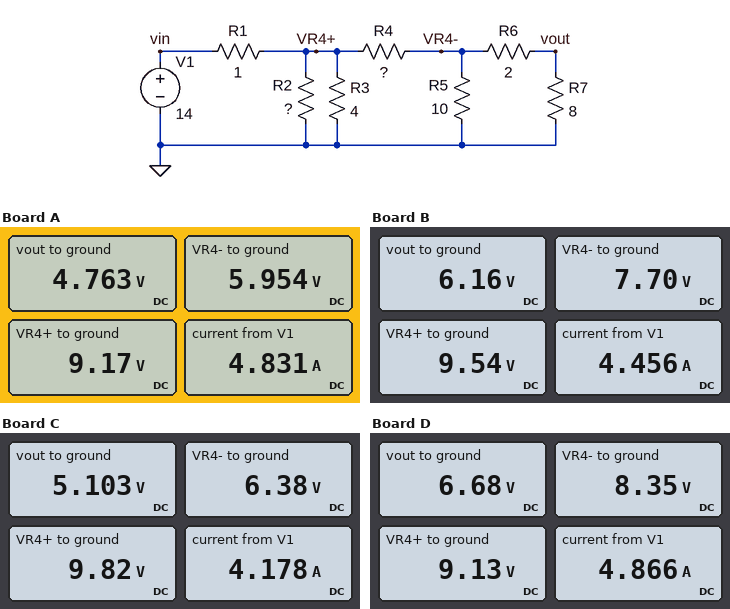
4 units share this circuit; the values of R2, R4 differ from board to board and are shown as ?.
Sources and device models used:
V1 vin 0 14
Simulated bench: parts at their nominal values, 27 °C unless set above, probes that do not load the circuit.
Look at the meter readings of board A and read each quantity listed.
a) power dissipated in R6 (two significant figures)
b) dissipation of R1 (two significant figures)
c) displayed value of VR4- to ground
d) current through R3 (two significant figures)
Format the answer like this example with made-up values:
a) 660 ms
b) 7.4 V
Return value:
a) 710 mW
b) 23 W
c) 5.954 V
d) 2.3 A
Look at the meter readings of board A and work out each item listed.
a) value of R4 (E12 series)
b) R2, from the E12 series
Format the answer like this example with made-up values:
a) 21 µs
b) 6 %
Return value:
a) 2.7 Ω
b) 6.8 Ω
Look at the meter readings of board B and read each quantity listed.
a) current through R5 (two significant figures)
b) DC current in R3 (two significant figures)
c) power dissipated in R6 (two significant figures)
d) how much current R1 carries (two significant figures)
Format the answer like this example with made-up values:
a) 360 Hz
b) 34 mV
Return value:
a) 770 mA
b) 2.4 A
c) 1.2 W
d) 4.5 A
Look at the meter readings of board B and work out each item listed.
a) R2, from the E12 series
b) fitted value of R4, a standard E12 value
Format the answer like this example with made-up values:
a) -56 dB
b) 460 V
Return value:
a) 18 Ω
b) 1.2 Ω
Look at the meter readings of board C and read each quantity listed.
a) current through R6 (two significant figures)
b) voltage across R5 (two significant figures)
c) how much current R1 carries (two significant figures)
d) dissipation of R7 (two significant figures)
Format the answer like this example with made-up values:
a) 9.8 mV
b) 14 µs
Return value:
a) 640 mA
b) 6.4 V
c) 4.2 A
d) 3.3 W
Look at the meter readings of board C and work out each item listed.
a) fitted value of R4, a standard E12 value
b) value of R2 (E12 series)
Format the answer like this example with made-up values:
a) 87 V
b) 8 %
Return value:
a) 2.7 Ω
b) 22 Ω
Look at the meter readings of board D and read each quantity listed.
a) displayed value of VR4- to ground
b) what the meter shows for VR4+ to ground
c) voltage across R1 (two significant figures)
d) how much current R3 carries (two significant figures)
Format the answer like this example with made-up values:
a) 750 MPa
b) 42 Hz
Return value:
a) 8.35 V
b) 9.13 V
c) 4.9 V
d) 2.3 A
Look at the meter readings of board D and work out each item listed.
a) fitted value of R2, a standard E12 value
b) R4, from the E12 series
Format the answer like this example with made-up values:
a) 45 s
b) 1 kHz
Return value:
a) 10 Ω
b) 0.47 Ω
